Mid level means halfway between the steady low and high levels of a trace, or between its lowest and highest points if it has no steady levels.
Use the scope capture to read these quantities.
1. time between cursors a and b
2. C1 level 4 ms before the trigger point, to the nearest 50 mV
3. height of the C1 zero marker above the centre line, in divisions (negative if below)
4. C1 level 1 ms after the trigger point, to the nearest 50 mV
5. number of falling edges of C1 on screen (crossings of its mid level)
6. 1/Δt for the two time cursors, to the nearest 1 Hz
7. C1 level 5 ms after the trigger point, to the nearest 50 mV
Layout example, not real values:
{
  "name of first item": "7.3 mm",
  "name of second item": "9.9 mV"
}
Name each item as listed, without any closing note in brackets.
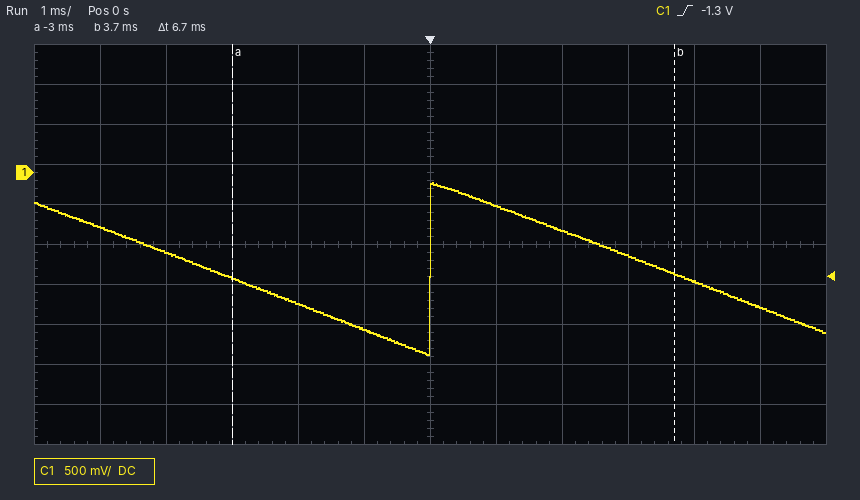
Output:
{
  "time between cursors a and b": "6.7 ms",
  "C1 level 4 ms before the trigger point, to the nearest 50 mV": "-1.00 V",
  "height of the C1 zero marker above the centre line, in divisions": "+1.8 div",
  "C1 level 1 ms after the trigger point, to the nearest 50 mV": "-400 mV",
  "number of falling edges of C1 on screen": "2",
  "1/Δt for the two time cursors, to the nearest 1 Hz": "149 Hz",
  "C1 level 5 ms after the trigger point, to the nearest 50 mV": "-1.70 V"
}
